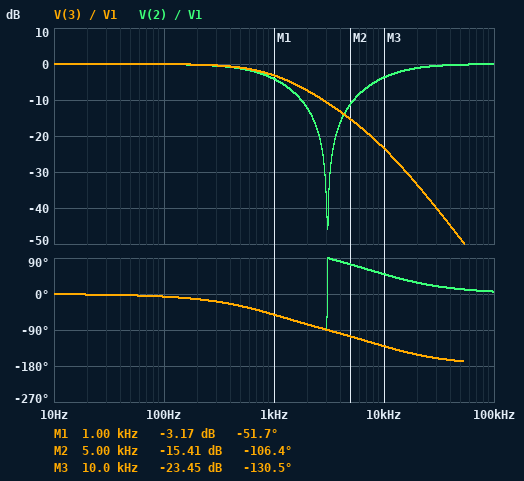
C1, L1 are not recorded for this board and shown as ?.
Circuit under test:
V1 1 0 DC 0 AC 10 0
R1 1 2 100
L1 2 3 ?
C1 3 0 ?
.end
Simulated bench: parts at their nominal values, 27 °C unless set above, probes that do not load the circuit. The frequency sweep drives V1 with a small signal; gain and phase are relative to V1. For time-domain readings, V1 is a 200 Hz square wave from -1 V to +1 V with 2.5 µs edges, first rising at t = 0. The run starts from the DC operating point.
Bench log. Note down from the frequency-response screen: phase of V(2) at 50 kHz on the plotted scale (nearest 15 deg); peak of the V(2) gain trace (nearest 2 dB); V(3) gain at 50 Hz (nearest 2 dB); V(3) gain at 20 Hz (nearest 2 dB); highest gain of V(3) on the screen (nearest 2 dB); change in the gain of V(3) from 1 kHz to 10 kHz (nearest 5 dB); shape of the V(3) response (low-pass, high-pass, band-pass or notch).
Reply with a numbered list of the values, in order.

1. 15 deg
2. 0 dB
3. 0 dB
4. 0 dB
5. 0 dB
6. -20 dB
7. low-pass
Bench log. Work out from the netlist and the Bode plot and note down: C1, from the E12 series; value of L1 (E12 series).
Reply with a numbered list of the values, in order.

1. 1.8 µF
2. 1.5 mH
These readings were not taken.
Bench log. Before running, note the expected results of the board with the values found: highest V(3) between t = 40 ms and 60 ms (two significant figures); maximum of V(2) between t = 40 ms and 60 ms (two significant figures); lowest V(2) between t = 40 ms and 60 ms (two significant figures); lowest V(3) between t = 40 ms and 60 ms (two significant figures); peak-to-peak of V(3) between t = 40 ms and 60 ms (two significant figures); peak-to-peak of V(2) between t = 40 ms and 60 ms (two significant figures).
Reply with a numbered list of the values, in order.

1. 1.0 V
2. 1.0 V
3. -1.0 V
4. -1.0 V
5. 2.0 V
6. 2.0 V
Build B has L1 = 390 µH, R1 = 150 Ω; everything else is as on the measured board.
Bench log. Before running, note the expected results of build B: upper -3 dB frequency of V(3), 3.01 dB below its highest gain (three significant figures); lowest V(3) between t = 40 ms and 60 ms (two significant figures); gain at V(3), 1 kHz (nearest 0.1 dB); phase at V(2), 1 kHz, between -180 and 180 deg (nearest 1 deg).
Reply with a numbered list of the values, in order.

1. 595 Hz
2. -1.0 V
3. -5.8 dB
4. -60 deg
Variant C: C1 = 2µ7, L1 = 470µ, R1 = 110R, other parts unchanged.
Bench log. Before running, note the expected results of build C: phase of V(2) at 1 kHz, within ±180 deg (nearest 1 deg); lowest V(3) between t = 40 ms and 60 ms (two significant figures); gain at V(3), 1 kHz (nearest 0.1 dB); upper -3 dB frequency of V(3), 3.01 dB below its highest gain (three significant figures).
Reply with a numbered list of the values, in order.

1. -63 deg
2. -1.0 V
3. -6.4 dB
4. 544 Hz
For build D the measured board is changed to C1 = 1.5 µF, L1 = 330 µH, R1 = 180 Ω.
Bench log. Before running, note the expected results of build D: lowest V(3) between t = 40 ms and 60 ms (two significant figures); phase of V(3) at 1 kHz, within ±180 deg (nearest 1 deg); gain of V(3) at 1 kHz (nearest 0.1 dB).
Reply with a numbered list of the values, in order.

1. -1.0 V
2. -60 deg
3. -5.8 dB
